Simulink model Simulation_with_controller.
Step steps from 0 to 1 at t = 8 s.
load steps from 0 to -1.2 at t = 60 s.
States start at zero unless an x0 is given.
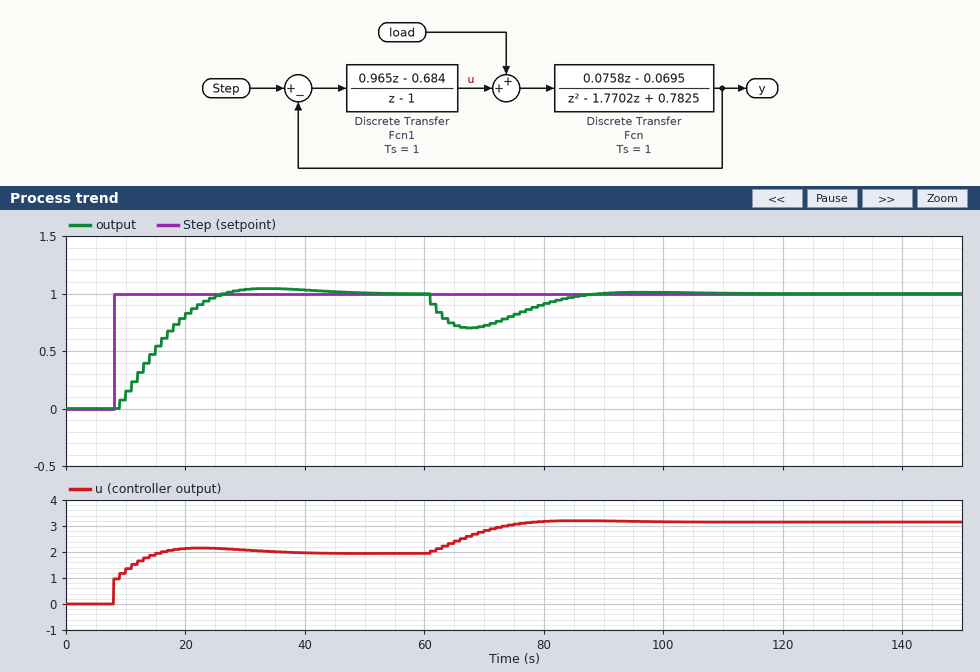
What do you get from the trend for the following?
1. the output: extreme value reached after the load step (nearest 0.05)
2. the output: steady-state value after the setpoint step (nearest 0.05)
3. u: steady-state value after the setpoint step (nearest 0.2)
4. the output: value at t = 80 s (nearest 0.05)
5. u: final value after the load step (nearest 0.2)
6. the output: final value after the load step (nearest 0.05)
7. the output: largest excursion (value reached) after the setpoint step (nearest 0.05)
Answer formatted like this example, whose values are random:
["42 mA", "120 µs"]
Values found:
["0.70", "1.00", "2.0", "0.90", "3.2", "1.00", "1.05"]
